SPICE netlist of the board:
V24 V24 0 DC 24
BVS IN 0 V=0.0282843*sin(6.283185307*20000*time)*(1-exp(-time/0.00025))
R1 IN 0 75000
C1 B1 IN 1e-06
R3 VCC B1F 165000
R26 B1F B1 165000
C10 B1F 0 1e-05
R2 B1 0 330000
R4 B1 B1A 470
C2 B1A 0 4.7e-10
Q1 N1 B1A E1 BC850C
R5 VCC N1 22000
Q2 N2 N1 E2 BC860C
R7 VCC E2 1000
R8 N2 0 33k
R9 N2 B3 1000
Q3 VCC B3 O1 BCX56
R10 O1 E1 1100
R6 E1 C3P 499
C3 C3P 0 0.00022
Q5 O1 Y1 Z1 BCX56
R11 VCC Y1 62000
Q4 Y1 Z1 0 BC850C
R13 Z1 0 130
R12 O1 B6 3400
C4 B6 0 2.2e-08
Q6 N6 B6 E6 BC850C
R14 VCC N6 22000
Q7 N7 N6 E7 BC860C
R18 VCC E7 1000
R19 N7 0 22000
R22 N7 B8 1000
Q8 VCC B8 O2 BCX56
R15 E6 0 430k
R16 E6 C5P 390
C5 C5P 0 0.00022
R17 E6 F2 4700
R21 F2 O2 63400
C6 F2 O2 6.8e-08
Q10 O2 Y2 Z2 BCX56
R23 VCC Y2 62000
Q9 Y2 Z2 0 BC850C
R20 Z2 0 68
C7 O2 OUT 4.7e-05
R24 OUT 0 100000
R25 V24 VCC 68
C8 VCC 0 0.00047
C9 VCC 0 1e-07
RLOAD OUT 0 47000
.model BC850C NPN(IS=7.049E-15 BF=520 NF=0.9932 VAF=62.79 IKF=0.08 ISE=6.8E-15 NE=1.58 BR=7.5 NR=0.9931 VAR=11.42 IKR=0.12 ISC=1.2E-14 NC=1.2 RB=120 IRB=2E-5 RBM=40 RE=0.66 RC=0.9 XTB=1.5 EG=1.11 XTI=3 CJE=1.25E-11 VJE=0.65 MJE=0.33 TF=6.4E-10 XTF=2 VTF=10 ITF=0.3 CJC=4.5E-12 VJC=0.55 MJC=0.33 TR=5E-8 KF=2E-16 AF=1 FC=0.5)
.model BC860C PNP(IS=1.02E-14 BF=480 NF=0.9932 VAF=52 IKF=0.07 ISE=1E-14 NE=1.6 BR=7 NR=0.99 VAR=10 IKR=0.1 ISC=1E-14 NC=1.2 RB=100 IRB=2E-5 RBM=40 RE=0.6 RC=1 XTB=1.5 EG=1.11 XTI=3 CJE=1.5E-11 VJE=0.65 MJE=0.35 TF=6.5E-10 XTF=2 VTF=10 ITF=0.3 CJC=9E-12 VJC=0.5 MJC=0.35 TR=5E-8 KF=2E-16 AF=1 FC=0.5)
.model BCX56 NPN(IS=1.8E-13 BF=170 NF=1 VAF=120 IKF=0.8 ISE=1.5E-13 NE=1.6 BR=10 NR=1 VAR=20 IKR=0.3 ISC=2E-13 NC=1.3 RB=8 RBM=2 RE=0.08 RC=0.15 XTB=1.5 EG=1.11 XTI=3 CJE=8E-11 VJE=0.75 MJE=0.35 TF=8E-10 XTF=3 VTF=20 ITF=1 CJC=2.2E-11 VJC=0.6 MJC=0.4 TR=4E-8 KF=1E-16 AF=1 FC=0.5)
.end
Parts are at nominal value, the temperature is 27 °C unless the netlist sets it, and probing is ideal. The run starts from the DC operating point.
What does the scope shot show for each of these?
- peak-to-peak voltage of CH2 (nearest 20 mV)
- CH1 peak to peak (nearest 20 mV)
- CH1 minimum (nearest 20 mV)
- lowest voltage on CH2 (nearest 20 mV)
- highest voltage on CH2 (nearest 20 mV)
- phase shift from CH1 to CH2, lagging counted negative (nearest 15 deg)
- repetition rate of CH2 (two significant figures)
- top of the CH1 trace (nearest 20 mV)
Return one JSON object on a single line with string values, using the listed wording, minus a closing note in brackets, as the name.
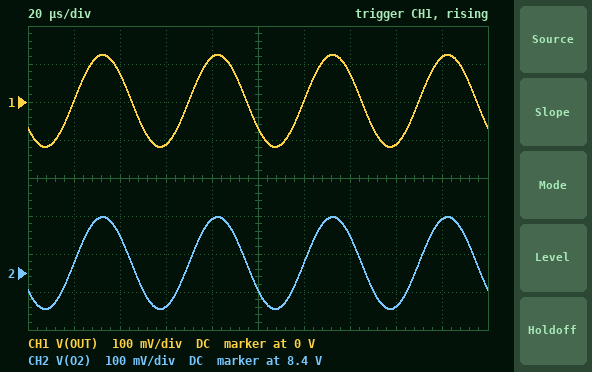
{"peak-to-peak voltage of CH2": "240 mV", "CH1 peak to peak": "240 mV", "CH1 minimum": "-120 mV", "lowest voltage on CH2": "8.30 V", "highest voltage on CH2": "8.54 V", "phase shift from CH1 to CH2, lagging counted negative": "0 deg", "repetition rate of CH2": "20 kHz", "top of the CH1 trace": "120 mV"}
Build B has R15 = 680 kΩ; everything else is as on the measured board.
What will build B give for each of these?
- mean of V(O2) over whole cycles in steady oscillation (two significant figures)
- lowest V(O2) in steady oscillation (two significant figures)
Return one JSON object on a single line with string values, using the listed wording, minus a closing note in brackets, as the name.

{"mean of V(O2) over whole cycles in steady oscillation": "7.9 V", "lowest V(O2) in steady oscillation": "7.8 V"}
